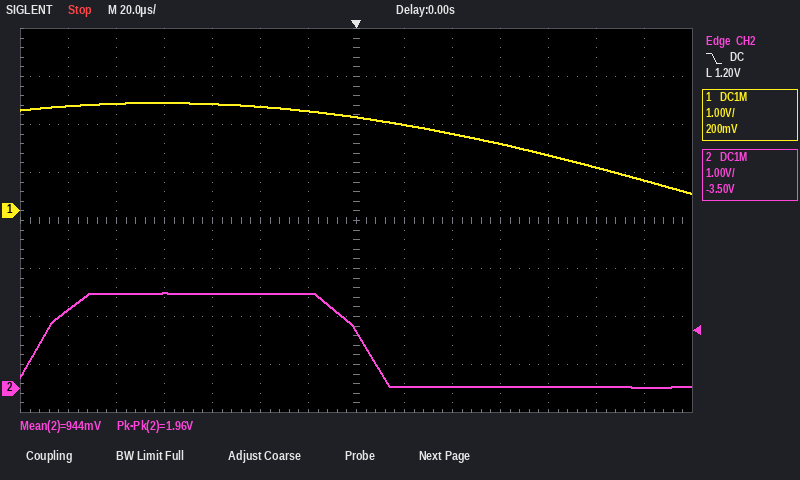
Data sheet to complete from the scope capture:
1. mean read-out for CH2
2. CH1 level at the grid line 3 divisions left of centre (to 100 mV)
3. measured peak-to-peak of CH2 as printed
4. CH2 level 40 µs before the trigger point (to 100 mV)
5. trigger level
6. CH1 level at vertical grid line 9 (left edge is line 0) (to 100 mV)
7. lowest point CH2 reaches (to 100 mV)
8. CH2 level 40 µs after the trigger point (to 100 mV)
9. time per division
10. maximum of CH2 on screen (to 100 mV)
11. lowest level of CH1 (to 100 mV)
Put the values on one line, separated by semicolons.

944 mV; 2.2 V; 1.96 V; 2.0 V; 1.20 V; 1.6 V; 0.0 V; 0.0 V; 20 µs; 2.0 V; 400 mV
